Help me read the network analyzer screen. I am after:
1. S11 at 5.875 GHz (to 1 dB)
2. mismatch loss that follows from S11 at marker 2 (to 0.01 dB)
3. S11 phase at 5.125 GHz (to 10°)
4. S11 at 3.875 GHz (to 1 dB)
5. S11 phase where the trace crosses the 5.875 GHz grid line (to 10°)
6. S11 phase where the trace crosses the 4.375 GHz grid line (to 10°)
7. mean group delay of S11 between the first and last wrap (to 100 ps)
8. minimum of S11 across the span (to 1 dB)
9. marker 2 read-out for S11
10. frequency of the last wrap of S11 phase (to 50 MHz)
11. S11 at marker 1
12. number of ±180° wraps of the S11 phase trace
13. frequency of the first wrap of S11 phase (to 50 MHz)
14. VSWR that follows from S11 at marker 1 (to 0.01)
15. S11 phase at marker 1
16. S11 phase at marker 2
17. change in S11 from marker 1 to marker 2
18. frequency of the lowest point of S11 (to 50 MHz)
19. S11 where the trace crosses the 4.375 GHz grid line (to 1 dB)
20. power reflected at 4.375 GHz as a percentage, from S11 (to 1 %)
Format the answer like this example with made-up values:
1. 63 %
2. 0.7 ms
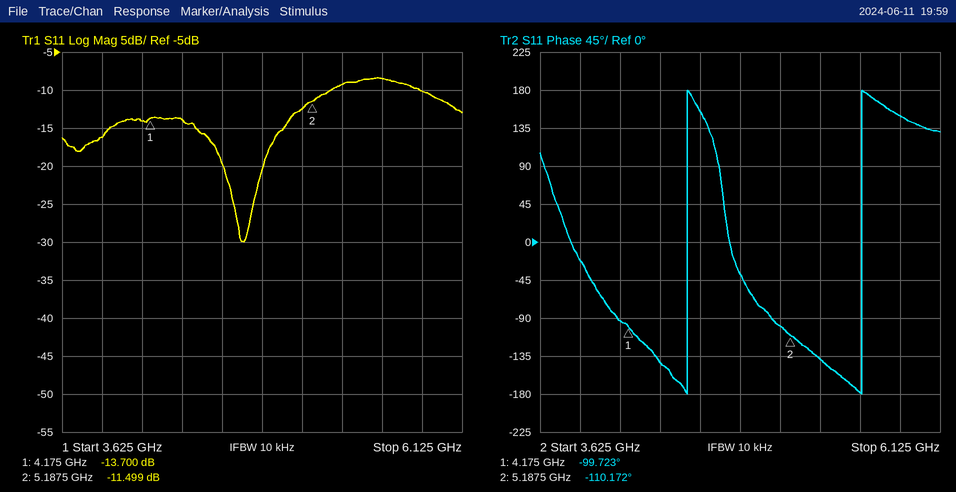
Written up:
1. -10 dB
2. 0.32 dB
3. -100°
4. -16 dB
5. 150°
6. -140°
7. 900 ps
8. -30 dB
9. -11.499 dB
10. 5.65 GHz
11. -13.700 dB
12. 2
13. 4.55 GHz
14. 1.52
15. -99.723°
16. -110.172°
17. 2.201 dB
18. 4.75 GHz
19. -14 dB
20. 4 %
